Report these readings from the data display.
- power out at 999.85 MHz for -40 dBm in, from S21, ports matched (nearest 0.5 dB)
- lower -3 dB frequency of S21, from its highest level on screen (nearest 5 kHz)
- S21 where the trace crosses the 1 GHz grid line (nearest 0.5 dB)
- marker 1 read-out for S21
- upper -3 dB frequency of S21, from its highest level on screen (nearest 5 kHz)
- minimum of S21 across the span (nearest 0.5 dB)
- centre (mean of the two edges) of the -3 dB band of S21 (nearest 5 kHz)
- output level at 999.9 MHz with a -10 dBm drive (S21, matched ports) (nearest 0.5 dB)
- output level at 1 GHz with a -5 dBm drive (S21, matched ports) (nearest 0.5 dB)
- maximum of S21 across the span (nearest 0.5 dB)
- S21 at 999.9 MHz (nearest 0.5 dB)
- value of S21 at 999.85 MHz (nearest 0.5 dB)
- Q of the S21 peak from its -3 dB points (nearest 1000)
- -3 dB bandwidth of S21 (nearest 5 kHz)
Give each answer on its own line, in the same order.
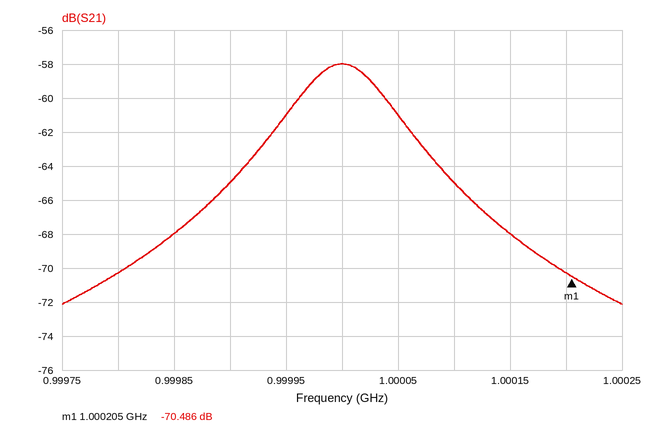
-108.0 dBm
999.950 MHz
-58.0 dB
-70.486 dB
1.000050 GHz
-72.0 dB
1.000000 GHz
-75.0 dBm
-63.0 dBm
-58.0 dB
-65.0 dB
-68.0 dB
10000
100 kHz
